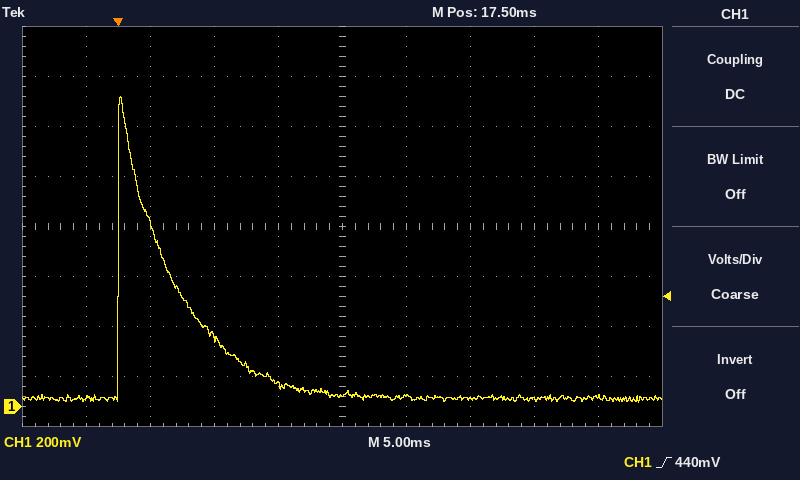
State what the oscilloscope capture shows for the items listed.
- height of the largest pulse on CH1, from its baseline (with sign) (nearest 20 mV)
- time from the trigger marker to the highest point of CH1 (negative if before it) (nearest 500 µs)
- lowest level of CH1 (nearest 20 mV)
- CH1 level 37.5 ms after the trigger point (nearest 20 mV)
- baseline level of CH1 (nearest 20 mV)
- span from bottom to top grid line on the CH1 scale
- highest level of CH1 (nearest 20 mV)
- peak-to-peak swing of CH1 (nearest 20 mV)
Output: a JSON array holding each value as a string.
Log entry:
["+1.20 V", "0.0 ms", "20 mV", "40 mV", "40 mV", "1.6 V", "1.24 V", "1.22 V"]
